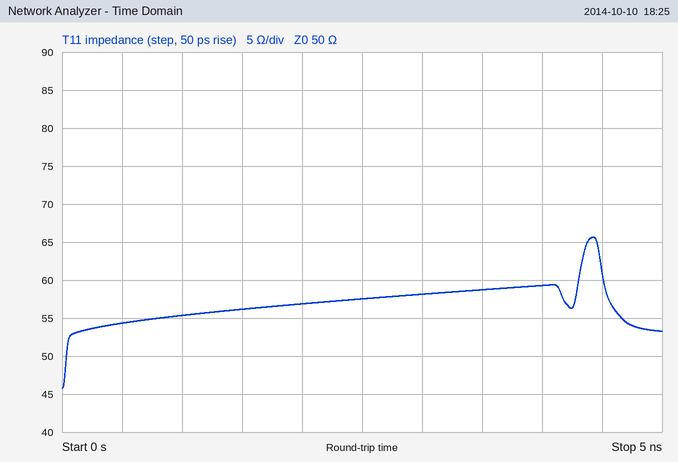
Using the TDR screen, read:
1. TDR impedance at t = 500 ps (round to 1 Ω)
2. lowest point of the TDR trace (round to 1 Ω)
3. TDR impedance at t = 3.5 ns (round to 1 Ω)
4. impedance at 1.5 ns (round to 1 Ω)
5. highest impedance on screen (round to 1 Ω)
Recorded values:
54 Ω
46 Ω
59 Ω
56 Ω
66 Ω
